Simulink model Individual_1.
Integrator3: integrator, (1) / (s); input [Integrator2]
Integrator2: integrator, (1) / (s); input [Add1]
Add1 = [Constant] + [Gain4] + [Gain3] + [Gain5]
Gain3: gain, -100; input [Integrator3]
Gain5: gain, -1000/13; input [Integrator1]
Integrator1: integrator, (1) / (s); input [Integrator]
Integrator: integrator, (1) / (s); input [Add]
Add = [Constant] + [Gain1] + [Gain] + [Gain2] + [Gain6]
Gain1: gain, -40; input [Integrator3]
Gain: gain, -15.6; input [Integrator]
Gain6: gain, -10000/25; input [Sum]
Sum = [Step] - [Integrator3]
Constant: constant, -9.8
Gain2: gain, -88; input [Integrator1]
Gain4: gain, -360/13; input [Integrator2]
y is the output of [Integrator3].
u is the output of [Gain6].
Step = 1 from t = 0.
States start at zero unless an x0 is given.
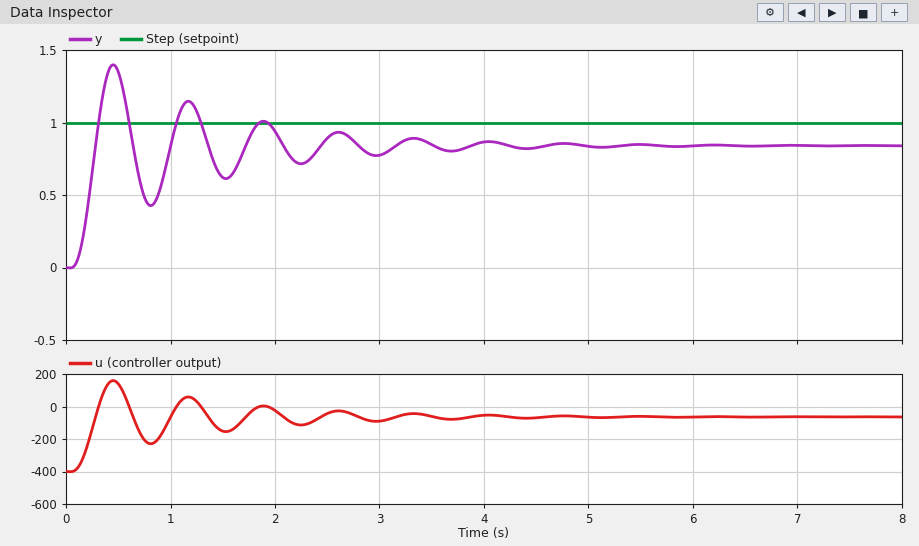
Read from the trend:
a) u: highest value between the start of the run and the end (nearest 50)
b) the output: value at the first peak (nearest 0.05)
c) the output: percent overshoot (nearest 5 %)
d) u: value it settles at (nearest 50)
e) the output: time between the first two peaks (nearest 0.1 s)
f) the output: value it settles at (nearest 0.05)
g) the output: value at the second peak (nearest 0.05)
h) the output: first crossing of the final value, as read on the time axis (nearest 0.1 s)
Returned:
150
1.40
65 %
-50
0.7 s
0.85
1.15
0.3 s
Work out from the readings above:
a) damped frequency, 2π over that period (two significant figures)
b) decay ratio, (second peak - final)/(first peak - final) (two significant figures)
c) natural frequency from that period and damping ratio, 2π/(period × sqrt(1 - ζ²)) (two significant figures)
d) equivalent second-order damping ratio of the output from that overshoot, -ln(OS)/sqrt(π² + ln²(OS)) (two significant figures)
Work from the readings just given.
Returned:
9.0 rad/s
0.55
9.1 rad/s
0.14
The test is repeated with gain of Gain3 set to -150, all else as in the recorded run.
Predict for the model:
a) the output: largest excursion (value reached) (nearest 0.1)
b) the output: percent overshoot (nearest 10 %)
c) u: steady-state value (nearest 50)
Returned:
1.2
60 %
-100
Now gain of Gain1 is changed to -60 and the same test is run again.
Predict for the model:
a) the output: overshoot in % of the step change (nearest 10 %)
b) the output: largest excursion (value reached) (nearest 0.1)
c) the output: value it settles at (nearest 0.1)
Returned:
60 %
1.4
0.9
